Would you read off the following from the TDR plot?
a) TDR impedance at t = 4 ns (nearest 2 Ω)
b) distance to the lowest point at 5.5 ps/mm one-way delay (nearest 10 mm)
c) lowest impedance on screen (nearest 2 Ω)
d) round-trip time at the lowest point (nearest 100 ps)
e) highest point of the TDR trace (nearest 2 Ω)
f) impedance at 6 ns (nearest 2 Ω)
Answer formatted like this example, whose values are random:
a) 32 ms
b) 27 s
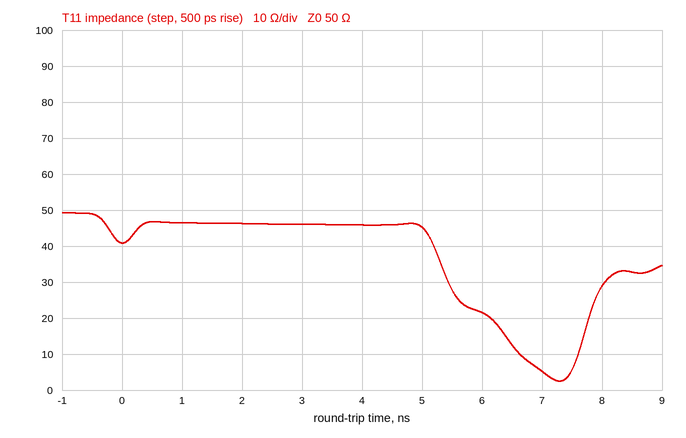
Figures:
a) 46 Ω
b) 660 mm
c) 2 Ω
d) 7.3 ns
e) 50 Ω
f) 22 Ω
